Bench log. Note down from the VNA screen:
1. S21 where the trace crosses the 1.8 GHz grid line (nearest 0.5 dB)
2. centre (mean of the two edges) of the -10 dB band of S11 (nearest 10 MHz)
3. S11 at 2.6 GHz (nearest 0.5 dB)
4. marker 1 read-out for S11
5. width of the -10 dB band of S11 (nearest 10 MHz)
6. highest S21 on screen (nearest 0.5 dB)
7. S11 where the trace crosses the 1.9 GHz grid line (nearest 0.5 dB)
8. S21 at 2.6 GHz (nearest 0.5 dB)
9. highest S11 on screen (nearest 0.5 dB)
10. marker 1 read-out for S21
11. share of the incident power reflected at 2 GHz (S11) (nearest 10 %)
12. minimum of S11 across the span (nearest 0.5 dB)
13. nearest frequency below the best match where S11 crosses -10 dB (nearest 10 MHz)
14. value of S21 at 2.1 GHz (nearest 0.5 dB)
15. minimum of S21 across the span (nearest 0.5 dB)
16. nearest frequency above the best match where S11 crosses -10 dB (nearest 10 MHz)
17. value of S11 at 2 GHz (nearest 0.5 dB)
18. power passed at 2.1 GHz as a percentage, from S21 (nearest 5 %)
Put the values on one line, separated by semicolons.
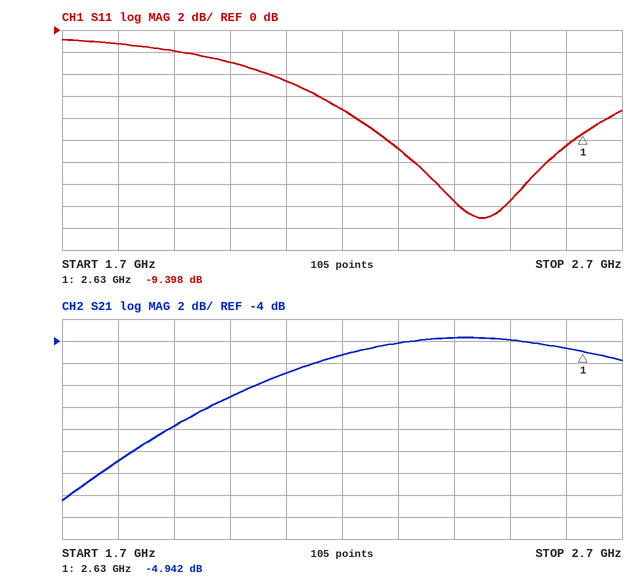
-15.0 dB; 2.45 GHz; -10.5 dB; -9.398 dB; 330 MHz; -3.5 dB; -2.0 dB; -4.5 dB; -1.0 dB; -4.942 dB; 50 %; -17.0 dB; 2.28 GHz; -7.0 dB; -18.5 dB; 2.61 GHz; -3.0 dB; 20 %
